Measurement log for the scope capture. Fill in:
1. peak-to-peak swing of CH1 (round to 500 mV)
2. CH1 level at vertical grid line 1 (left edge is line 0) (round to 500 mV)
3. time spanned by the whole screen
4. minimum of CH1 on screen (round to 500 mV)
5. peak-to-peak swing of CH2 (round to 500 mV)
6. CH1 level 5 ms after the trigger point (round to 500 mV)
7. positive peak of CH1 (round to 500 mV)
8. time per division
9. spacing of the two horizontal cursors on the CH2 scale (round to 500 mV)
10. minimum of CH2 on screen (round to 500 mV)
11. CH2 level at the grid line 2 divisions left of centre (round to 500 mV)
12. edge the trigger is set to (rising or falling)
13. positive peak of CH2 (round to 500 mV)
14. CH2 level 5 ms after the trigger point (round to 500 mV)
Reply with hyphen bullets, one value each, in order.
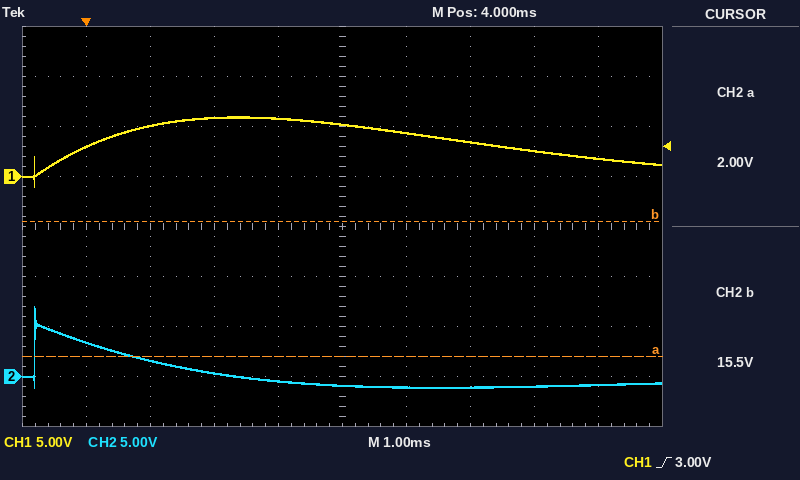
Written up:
- 7.0 V
- 3.0 V
- 10 ms
- -1.0 V
- 8.0 V
- 4.5 V
- 6.0 V
- 1 ms
- 13.5 V
- -1.0 V
- 500 mV
- rising
- 7.0 V
- -1.0 V
